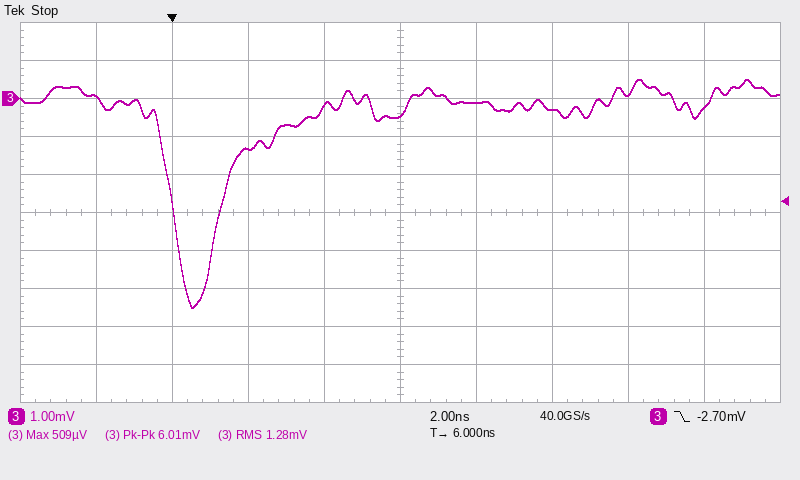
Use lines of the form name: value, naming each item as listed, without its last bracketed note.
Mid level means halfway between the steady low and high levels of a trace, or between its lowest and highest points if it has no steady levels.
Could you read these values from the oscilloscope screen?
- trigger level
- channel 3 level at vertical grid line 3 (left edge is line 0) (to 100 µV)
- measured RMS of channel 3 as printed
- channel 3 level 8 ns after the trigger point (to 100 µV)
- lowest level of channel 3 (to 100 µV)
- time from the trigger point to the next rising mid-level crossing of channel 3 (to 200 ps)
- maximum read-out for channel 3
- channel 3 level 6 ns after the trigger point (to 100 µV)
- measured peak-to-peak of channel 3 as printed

trigger level: -2.70 mV
channel 3 level at vertical grid line 3 (left edge is line 0): -1.3 mV
measured RMS of channel 3 as printed: 1.28 mV
channel 3 level 8 ns after the trigger point: -100 µV
lowest level of channel 3: -5.5 mV
time from the trigger point to the next rising mid-level crossing of channel 3: 1.4 ns
maximum read-out for channel 3: 509 µV
channel 3 level 6 ns after the trigger point: -400 µV
measured peak-to-peak of channel 3 as printed: 6.01 mV
